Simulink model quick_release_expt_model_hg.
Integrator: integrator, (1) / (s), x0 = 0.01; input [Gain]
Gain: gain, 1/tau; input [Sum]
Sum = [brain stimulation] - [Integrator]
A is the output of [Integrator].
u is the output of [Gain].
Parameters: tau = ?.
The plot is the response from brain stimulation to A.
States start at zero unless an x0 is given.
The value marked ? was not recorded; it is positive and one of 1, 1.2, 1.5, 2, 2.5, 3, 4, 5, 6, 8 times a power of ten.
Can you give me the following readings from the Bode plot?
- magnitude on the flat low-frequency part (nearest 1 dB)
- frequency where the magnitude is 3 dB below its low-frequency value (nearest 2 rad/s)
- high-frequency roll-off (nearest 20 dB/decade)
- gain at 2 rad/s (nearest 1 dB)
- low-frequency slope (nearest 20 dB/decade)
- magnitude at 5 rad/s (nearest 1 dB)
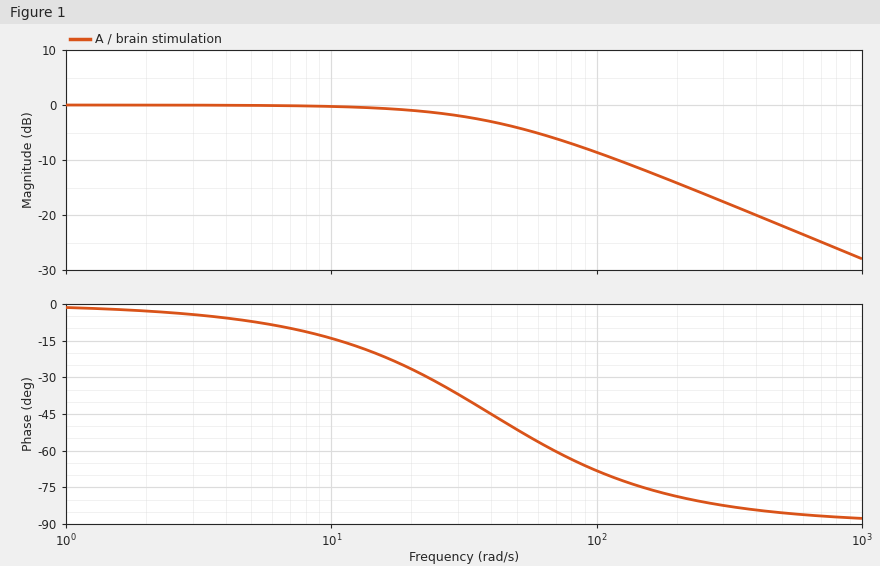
0 dB
40 rad/s
-20 dB/decade
0 dB
0 dB/decade
0 dB
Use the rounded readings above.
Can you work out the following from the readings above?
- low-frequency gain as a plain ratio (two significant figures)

1.0
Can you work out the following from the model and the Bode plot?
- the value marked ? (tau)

0.025
